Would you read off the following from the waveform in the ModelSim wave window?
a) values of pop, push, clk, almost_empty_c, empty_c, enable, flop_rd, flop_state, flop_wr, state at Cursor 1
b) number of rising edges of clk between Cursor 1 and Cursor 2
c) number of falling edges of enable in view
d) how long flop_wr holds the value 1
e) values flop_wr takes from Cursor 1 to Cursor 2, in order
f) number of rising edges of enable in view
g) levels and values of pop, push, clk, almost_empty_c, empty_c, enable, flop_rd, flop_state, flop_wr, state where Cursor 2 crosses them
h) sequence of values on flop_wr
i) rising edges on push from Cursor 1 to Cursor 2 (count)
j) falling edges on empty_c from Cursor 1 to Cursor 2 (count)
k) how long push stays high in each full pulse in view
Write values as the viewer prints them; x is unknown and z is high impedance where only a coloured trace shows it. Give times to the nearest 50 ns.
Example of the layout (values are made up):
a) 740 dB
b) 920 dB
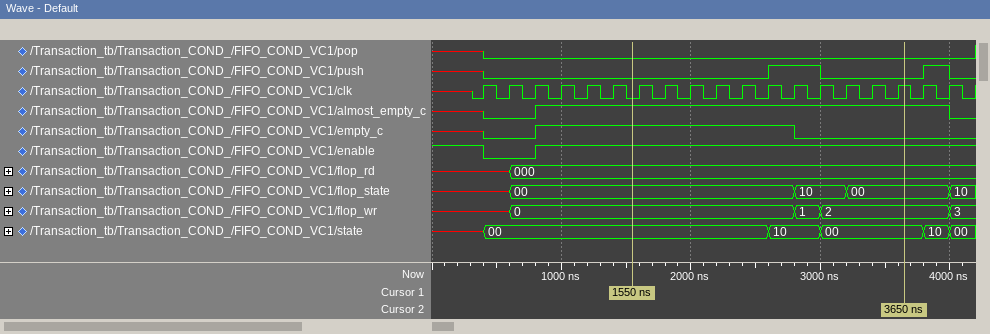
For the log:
a) pop=0, push=0, clk=0, almost_empty_c=1, empty_c=1, enable=1, flop_rd=000, flop_state=00, flop_wr=0, state=00
b) 11
c) 1
d) 200 ns
e) 0, 1, 2
f) 1
g) pop=0, push=0, clk=1, almost_empty_c=1, empty_c=0, enable=1, flop_rd=000, flop_state=00, flop_wr=2, state=00
h) x, 0, 1, 2, 3
i) 1
j) 1
k) 400 ns, 200 ns
